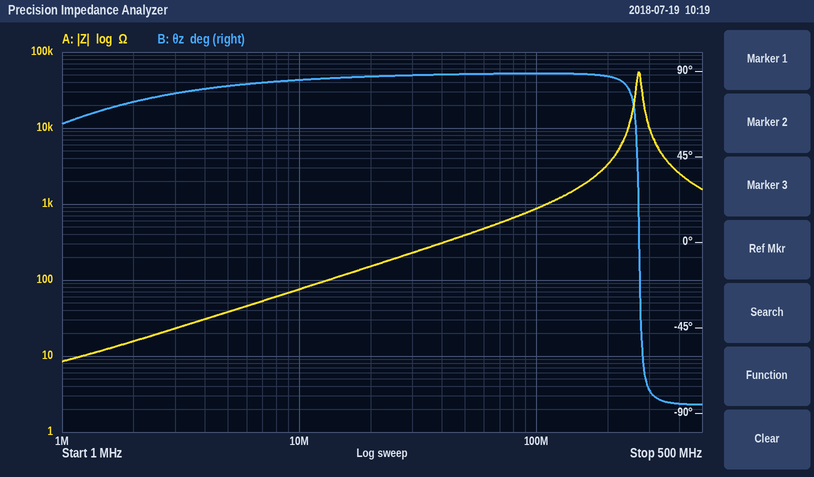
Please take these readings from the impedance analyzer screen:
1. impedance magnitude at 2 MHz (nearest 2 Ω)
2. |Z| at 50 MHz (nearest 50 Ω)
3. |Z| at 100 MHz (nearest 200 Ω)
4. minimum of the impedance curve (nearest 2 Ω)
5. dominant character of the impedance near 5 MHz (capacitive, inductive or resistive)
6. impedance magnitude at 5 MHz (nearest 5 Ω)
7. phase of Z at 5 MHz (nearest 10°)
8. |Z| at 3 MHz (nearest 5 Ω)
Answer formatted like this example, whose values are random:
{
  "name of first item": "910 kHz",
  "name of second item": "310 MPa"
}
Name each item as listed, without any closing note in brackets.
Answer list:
{
  "impedance magnitude at 2 MHz": "16 Ω",
  "|Z| at 50 MHz": "400 Ω",
  "|Z| at 100 MHz": "800 Ω",
  "minimum of the impedance curve": "8 Ω",
  "dominant character of the impedance near 5 MHz": "inductive",
  "impedance magnitude at 5 MHz": "40 Ω",
  "phase of Z at 5 MHz": "80°",
  "|Z| at 3 MHz": "25 Ω"
}
